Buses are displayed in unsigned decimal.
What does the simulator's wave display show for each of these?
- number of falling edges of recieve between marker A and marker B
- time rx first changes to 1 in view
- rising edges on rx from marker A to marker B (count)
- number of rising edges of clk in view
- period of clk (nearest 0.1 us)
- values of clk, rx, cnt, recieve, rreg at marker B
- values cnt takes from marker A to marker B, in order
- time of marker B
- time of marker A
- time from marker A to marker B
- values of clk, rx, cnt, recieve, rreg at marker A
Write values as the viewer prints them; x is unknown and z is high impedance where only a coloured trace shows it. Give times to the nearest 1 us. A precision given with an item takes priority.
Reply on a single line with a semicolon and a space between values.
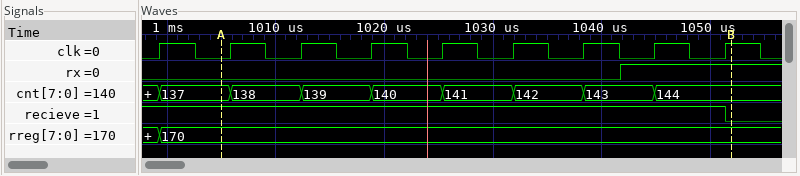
1; 1042 us; 1; 9; 6.5 us; clk=1, rx=1, cnt=144, recieve=0, rreg=170; 137, 138, 139, 140, 141, 142, 143, 144; 1052 us; 1005 us; 47 us; clk=0, rx=0, cnt=137, recieve=1, rreg=170
